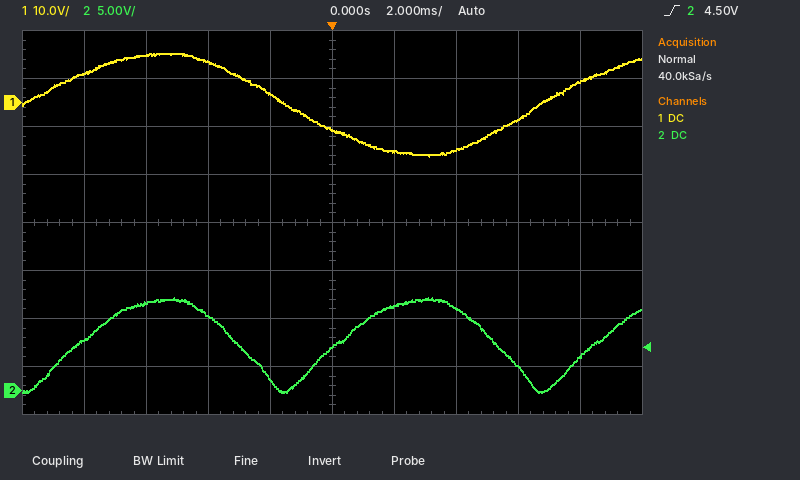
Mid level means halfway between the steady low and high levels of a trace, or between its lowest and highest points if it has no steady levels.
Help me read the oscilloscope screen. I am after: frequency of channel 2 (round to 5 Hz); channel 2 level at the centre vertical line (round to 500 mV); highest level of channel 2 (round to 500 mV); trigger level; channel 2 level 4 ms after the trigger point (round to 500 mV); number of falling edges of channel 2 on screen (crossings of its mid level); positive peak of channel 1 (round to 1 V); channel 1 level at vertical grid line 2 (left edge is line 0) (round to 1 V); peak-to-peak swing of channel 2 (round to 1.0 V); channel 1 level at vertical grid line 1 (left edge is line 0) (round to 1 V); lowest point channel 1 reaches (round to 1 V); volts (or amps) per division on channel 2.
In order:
120 Hz
4.5 V
9.5 V
4.50 V
8.5 V
2
10 V
10 V
10.0 V
6 V
-11 V
5 V
